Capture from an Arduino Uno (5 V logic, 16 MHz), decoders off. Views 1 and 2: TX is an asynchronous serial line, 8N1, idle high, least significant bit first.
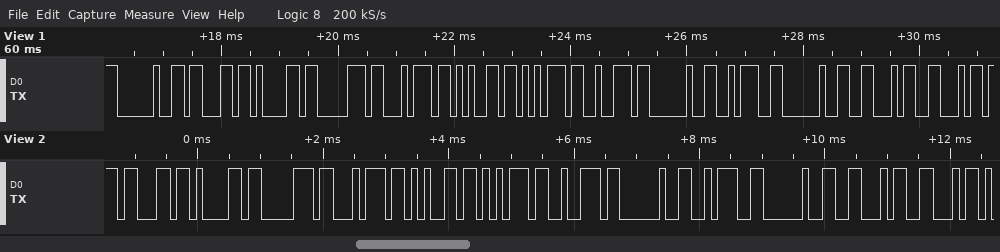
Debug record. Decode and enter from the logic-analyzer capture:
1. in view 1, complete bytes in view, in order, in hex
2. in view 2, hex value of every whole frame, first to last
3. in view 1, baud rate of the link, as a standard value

20 63 61 70 74 65 75 72 20 3A 20 46 46
63 61 70 74 65 75 72 20 3A 20 46 46
9600 baud
